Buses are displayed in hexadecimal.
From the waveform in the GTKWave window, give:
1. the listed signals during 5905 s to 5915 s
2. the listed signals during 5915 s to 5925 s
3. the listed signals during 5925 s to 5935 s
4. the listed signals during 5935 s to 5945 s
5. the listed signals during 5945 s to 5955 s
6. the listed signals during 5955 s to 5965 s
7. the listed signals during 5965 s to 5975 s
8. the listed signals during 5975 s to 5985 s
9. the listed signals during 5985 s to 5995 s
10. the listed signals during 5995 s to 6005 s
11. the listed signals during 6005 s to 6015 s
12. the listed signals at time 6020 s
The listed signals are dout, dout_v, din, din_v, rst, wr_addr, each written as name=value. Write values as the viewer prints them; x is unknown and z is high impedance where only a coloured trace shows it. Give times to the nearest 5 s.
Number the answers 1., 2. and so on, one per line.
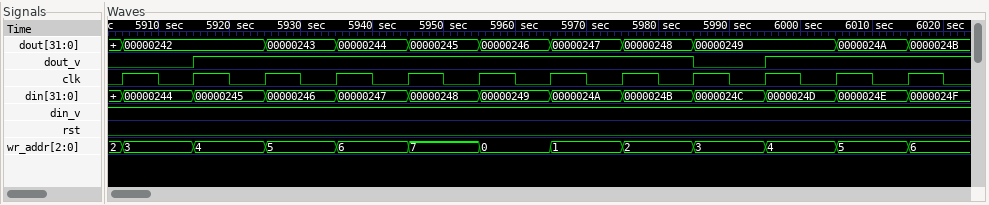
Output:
1. dout=00000242, dout_v=0, din=00000244, din_v=1, rst=0, wr_addr=3
2. dout=00000242, dout_v=1, din=00000245, din_v=1, rst=0, wr_addr=4
3. dout=00000243, dout_v=1, din=00000246, din_v=1, rst=0, wr_addr=5
4. dout=00000244, dout_v=1, din=00000247, din_v=1, rst=0, wr_addr=6
5. dout=00000245, dout_v=1, din=00000248, din_v=1, rst=0, wr_addr=7
6. dout=00000246, dout_v=1, din=00000249, din_v=1, rst=0, wr_addr=0
7. dout=00000247, dout_v=1, din=0000024A, din_v=1, rst=0, wr_addr=1
8. dout=00000248, dout_v=1, din=0000024B, din_v=1, rst=0, wr_addr=2
9. dout=00000249, dout_v=0, din=0000024C, din_v=1, rst=0, wr_addr=3
10. dout=00000249, dout_v=1, din=0000024D, din_v=1, rst=0, wr_addr=4
11. dout=0000024A, dout_v=1, din=0000024E, din_v=1, rst=0, wr_addr=5
12. dout=0000024B, dout_v=1, din=0000024F, din_v=1, rst=0, wr_addr=6
